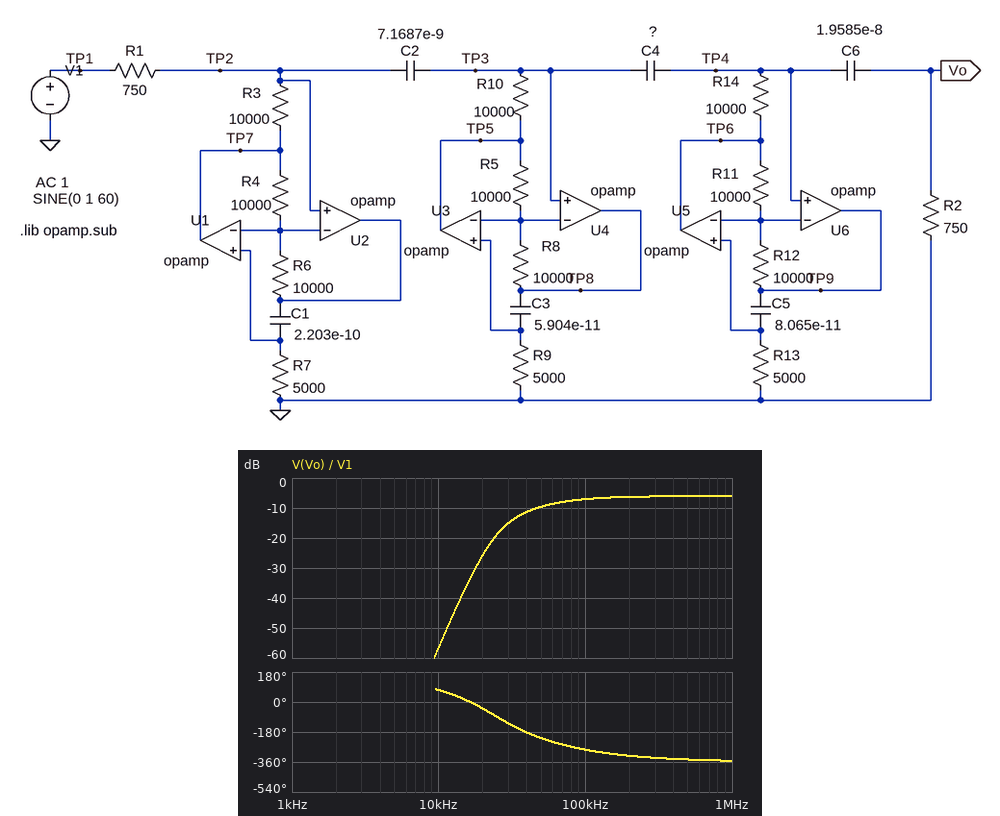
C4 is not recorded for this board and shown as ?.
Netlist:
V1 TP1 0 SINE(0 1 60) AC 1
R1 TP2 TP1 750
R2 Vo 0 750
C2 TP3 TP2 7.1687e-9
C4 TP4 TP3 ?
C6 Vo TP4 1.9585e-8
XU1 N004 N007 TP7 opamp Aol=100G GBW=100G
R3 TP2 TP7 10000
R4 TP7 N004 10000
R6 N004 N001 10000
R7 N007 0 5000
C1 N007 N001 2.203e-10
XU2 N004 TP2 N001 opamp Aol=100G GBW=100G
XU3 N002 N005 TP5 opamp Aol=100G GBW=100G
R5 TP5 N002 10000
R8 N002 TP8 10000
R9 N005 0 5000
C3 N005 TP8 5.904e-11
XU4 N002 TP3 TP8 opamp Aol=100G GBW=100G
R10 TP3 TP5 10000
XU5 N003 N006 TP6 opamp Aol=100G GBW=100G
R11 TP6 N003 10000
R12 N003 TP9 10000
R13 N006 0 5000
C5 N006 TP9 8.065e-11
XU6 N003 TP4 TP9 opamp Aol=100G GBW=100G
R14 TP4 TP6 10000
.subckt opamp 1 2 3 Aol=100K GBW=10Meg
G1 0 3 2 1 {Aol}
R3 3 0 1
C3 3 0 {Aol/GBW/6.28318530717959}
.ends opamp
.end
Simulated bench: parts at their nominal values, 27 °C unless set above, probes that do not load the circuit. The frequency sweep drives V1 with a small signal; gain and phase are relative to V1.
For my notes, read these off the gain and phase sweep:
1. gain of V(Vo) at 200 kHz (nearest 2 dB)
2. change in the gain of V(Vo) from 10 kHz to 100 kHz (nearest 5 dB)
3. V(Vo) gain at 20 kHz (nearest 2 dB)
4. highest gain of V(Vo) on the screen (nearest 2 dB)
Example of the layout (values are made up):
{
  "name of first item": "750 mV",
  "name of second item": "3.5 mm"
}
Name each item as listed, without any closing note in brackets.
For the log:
{
  "gain of V(Vo) at 200 kHz": "-6 dB",
  "change in the gain of V(Vo) from 10 kHz to 100 kHz": "50 dB",
  "V(Vo) gain at 20 kHz": "-26 dB",
  "highest gain of V(Vo) on the screen": "-6 dB"
}
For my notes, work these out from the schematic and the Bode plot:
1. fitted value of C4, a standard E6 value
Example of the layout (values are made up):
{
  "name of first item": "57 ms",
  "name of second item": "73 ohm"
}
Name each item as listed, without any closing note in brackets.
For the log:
{
  "fitted value of C4, a standard E6 value": "1.5 nF"
}
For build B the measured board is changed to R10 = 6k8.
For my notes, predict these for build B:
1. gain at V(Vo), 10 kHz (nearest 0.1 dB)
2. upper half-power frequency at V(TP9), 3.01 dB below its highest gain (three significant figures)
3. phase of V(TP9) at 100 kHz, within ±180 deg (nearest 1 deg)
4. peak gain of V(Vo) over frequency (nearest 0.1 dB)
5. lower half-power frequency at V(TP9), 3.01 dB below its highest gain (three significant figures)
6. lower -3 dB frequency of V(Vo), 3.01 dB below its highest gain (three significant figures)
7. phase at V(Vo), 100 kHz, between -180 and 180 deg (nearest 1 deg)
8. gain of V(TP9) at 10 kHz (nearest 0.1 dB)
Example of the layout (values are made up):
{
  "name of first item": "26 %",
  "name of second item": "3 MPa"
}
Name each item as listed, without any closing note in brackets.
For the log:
{
  "gain at V(Vo), 10 kHz": "-60.2 dB",
  "upper half-power frequency at V(TP9), 3.01 dB below its highest gain": "108 kHz",
  "phase of V(TP9) at 100 kHz, within ±180 deg": "0 deg",
  "peak gain of V(Vo) over frequency": "-6.0 dB",
  "lower half-power frequency at V(TP9), 3.01 dB below its highest gain": "30.9 kHz",
  "lower -3 dB frequency of V(Vo), 3.01 dB below its highest gain": "58.7 kHz",
  "phase at V(Vo), 100 kHz, between -180 and 180 deg": "82 deg",
  "gain of V(TP9) at 10 kHz": "-24.9 dB"
}
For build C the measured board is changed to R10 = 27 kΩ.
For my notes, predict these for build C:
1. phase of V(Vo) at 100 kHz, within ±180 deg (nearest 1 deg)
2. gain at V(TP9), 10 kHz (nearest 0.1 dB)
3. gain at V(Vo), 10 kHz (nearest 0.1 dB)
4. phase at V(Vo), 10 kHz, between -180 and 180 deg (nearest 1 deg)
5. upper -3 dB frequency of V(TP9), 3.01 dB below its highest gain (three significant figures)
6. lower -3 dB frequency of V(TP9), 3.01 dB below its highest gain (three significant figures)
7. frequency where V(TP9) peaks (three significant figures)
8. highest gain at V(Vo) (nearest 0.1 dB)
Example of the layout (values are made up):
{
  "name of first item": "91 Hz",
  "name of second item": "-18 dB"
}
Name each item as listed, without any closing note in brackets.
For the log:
{
  "phase of V(Vo) at 100 kHz, within ±180 deg": "64 deg",
  "gain at V(TP9), 10 kHz": "-10.5 dB",
  "gain at V(Vo), 10 kHz": "-45.8 dB",
  "phase at V(Vo), 10 kHz, between -180 and 180 deg": "69 deg",
  "upper -3 dB frequency of V(TP9), 3.01 dB below its highest gain": "54.7 kHz",
  "lower -3 dB frequency of V(TP9), 3.01 dB below its highest gain": "15.4 kHz",
  "frequency where V(TP9) peaks": "19.0 kHz",
  "highest gain at V(Vo)": "-6.0 dB"
}
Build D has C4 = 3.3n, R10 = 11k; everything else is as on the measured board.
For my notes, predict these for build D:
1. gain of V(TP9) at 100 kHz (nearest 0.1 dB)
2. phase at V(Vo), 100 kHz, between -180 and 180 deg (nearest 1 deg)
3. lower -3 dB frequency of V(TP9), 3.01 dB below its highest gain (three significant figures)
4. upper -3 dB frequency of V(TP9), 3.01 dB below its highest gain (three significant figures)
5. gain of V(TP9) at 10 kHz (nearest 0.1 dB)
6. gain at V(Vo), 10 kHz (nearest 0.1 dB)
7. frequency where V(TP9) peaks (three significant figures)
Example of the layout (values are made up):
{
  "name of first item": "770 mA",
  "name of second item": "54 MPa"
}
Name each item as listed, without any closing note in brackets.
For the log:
{
  "gain of V(TP9) at 100 kHz": "6.1 dB",
  "phase at V(Vo), 100 kHz, between -180 and 180 deg": "52 deg",
  "lower -3 dB frequency of V(TP9), 3.01 dB below its highest gain": "20.8 kHz",
  "upper -3 dB frequency of V(TP9), 3.01 dB below its highest gain": "45.1 kHz",
  "gain of V(TP9) at 10 kHz": "-12.9 dB",
  "gain at V(Vo), 10 kHz": "-48.2 dB",
  "frequency where V(TP9) peaks": "27.3 kHz"
}
